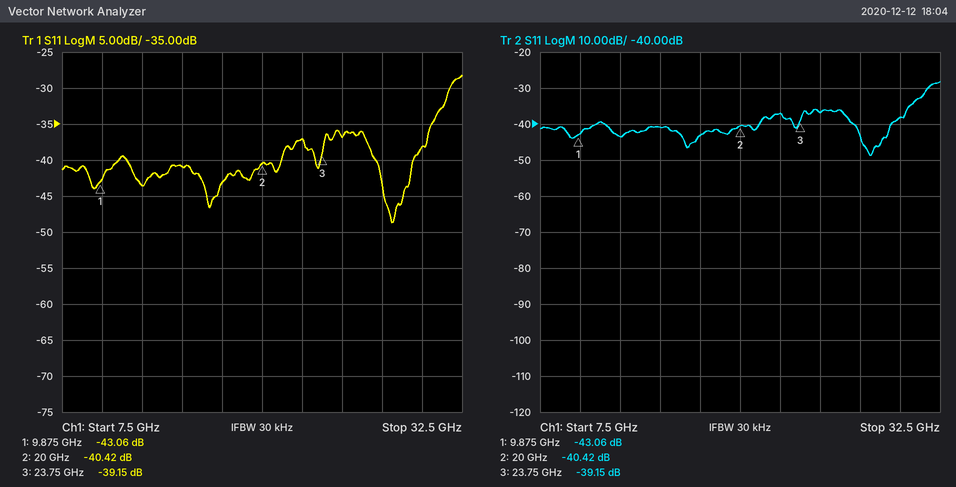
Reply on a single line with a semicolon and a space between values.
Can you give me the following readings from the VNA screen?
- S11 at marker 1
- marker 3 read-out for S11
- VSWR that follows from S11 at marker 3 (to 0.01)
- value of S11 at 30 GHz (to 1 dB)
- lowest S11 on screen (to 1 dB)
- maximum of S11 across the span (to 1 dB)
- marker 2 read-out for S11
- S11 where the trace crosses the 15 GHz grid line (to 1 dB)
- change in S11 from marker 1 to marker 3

-43.06 dB; -39.15 dB; 1.02; -38 dB; -49 dB; -28 dB; -40.42 dB; -41 dB; 3.91 dB
